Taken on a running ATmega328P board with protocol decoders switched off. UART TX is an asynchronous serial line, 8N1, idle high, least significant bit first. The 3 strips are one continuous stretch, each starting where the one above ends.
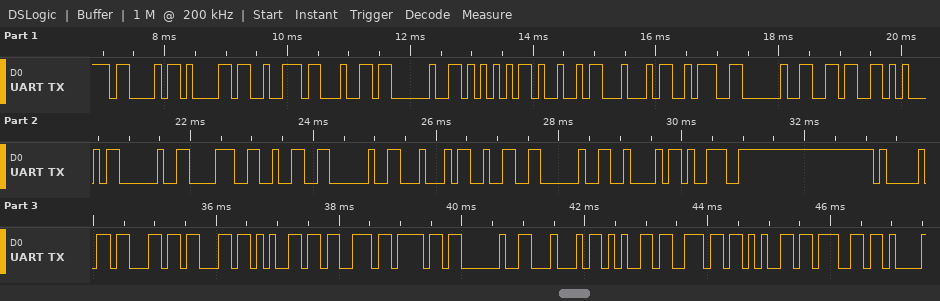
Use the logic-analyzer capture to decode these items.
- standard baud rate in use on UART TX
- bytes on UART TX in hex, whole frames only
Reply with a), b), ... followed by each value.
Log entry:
a) 9600 baud
b) 43 61 72 64 20 55 49 44 3A 20 36 45 20 38 32 20 44 32 20 42 39 41 63 63 65 73 6F 20 44 65 6E 65 67
